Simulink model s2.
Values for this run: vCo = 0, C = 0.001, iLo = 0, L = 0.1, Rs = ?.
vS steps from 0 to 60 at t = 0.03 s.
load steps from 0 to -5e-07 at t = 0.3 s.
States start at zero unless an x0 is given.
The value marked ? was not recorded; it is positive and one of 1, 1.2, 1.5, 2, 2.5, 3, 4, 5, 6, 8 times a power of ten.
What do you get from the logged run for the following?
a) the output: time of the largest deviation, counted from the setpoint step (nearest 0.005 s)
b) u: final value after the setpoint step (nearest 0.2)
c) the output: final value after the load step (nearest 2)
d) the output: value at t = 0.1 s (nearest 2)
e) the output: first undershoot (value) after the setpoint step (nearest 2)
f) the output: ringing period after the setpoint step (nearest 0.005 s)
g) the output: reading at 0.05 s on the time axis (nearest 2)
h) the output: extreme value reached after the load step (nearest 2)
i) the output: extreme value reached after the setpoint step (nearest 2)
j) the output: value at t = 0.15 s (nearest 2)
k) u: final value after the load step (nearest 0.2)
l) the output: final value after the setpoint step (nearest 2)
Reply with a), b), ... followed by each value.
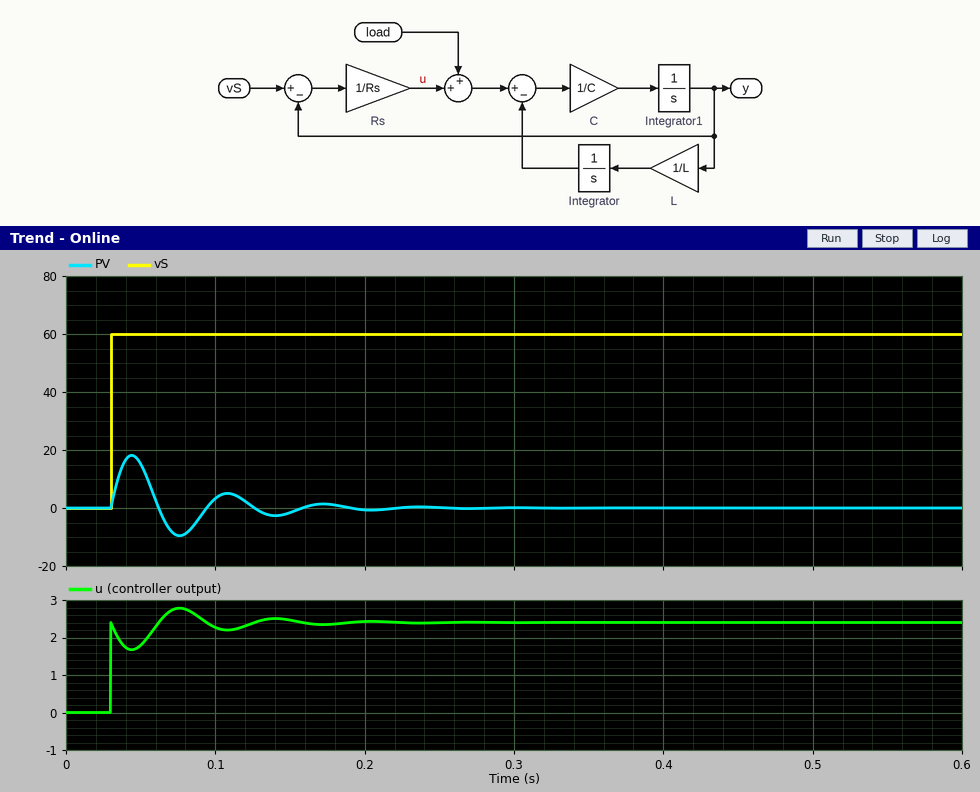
a) 0.015 s
b) 2.4
c) 0
d) 4
e) -10
f) 0.065 s
g) 16
h) 0
i) 18
j) -2
k) 2.4
l) 0
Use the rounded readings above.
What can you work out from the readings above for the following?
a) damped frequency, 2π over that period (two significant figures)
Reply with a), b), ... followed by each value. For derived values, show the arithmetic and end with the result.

a) 2π / 0.065 = 97 rad/s
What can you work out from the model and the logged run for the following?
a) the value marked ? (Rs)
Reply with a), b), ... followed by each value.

a) 25
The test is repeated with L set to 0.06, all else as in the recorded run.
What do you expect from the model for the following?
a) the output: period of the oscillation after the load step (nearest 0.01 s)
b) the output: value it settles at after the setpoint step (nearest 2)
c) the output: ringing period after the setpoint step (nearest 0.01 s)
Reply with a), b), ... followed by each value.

a) 0.05 s
b) 0
c) 0.05 s
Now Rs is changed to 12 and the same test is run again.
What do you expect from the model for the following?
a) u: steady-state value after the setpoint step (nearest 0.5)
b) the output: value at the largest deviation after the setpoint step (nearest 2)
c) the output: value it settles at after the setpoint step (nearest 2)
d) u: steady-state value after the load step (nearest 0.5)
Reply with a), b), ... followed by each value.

a) 5.0
b) 30
c) 0
d) 5.0
